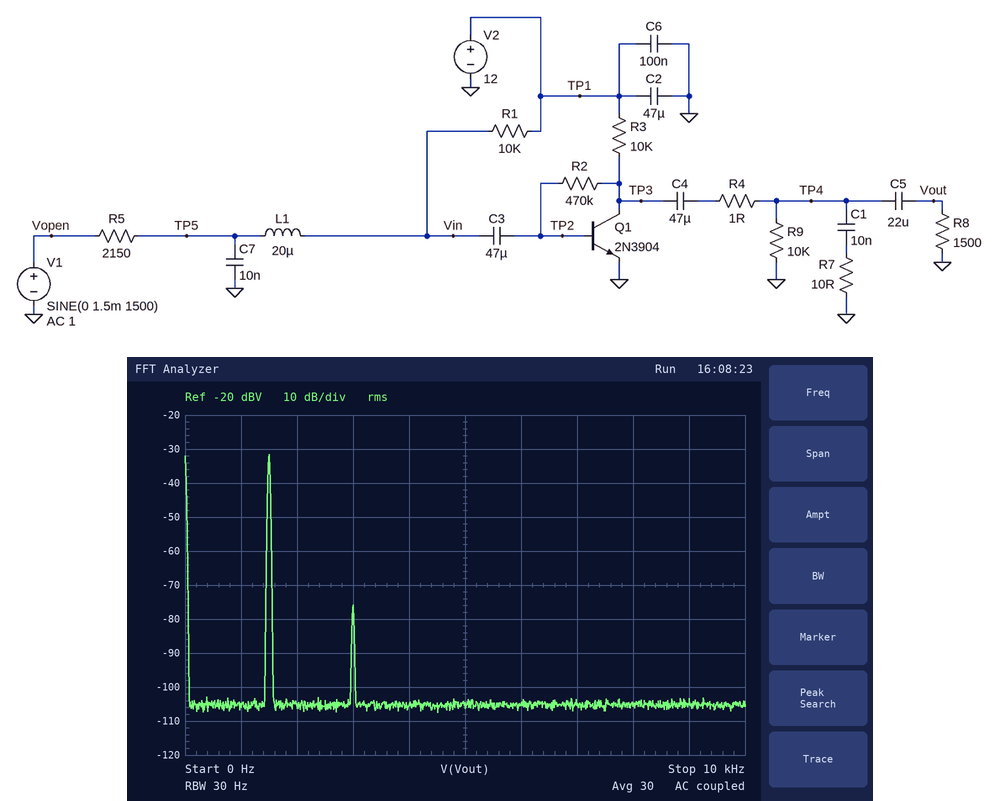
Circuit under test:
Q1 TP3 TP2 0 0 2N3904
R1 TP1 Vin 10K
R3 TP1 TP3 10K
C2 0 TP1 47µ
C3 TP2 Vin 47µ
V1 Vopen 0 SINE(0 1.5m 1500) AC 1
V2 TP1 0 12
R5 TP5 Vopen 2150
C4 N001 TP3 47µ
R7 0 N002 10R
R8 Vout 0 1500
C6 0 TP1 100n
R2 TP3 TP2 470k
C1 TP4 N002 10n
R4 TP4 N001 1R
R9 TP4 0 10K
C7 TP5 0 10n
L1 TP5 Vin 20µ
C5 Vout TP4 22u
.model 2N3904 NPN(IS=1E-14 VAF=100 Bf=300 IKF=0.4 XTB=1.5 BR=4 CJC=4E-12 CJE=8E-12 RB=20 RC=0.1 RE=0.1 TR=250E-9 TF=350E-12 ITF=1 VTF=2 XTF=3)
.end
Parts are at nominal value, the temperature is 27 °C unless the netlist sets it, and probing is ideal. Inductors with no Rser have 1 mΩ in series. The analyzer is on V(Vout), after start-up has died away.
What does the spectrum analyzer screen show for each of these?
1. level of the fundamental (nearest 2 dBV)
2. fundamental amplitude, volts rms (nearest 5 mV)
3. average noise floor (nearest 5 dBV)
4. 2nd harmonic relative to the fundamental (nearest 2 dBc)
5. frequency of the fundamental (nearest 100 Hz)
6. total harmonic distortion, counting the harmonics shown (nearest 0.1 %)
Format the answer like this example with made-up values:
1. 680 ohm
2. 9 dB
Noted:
1. -32 dBV
2. 25 mV
3. -105 dBV
4. -44 dBc
5. 1.5 kHz
6. 0.6 %
